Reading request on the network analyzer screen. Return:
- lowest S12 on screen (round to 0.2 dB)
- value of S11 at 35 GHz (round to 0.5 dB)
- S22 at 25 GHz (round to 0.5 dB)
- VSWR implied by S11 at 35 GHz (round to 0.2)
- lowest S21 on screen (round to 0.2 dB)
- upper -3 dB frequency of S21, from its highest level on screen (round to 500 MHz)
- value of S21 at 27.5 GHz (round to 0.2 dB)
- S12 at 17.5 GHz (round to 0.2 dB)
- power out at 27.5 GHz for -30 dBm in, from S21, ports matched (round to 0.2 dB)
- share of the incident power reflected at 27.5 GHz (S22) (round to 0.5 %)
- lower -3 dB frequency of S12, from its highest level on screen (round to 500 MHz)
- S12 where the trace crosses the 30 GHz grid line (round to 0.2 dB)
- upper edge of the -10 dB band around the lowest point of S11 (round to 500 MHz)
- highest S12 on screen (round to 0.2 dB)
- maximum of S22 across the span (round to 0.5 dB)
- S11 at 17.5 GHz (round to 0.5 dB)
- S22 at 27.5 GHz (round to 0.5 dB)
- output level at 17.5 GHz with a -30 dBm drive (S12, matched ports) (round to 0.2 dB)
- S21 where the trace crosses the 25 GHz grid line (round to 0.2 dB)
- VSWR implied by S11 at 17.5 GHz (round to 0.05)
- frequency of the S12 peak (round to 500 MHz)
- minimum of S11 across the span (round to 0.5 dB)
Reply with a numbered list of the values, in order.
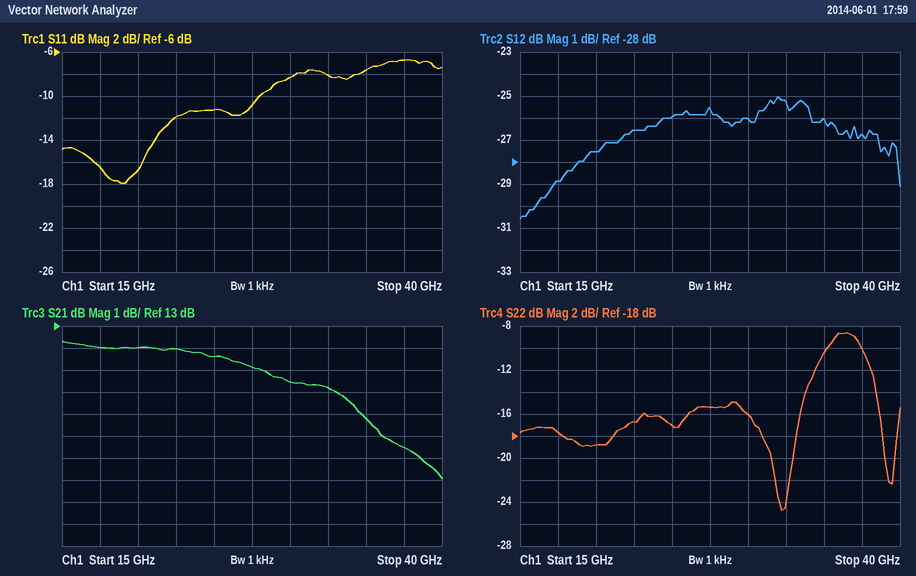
1. -30.6 dB
2. -7.5 dB
3. -17.0 dB
4. 2.4
5. 6.0 dB
6. 34.5 GHz
7. 11.2 dB
8. -28.8 dB
9. -18.8 dBm
10. 3.0 %
11. 19.0 GHz
12. -26.0 dB
13. 28.0 GHz
14. -25.0 dB
15. -8.5 dB
16. -16.5 dB
17. -15.5 dB
18. -58.8 dBm
19. 11.6 dB
20. 1.35
21. 32.0 GHz
22. -18.0 dB
